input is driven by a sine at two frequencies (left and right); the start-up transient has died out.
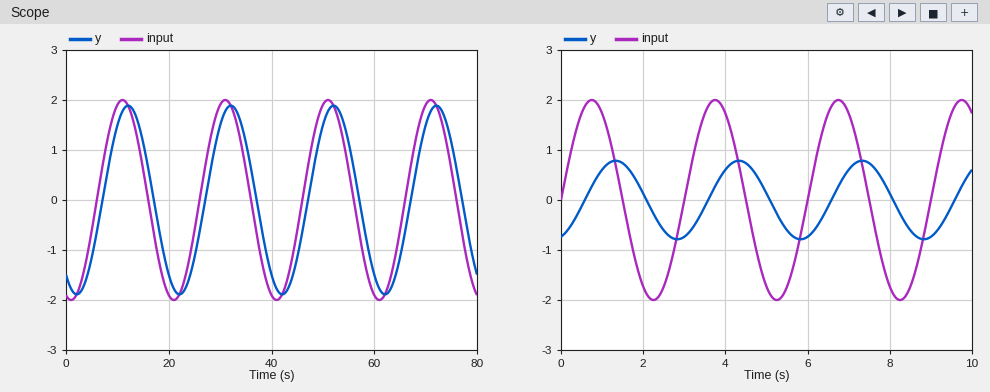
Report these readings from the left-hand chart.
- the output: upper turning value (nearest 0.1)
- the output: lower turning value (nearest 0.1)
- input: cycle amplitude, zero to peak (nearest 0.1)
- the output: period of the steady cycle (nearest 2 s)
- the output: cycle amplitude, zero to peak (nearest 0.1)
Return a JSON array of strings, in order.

["1.9", "-1.9", "2.0", "20 s", "1.9"]
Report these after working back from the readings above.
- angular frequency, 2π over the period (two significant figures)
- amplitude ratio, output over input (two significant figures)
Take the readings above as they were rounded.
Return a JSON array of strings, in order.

["0.31 rad/s", "0.95"]
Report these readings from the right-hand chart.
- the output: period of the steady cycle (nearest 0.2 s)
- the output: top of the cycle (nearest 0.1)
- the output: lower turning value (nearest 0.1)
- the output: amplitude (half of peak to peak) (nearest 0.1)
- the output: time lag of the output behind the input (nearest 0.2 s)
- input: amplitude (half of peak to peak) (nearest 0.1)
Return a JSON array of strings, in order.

["3.0 s", "0.8", "-0.8", "0.8", "0.6 s", "2.0"]
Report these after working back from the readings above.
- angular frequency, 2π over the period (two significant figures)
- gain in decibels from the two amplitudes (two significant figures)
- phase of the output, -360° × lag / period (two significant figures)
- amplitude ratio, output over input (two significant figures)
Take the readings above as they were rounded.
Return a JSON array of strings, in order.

["2.1 rad/s", "-8.0 dB", "-72°", "0.40"]
